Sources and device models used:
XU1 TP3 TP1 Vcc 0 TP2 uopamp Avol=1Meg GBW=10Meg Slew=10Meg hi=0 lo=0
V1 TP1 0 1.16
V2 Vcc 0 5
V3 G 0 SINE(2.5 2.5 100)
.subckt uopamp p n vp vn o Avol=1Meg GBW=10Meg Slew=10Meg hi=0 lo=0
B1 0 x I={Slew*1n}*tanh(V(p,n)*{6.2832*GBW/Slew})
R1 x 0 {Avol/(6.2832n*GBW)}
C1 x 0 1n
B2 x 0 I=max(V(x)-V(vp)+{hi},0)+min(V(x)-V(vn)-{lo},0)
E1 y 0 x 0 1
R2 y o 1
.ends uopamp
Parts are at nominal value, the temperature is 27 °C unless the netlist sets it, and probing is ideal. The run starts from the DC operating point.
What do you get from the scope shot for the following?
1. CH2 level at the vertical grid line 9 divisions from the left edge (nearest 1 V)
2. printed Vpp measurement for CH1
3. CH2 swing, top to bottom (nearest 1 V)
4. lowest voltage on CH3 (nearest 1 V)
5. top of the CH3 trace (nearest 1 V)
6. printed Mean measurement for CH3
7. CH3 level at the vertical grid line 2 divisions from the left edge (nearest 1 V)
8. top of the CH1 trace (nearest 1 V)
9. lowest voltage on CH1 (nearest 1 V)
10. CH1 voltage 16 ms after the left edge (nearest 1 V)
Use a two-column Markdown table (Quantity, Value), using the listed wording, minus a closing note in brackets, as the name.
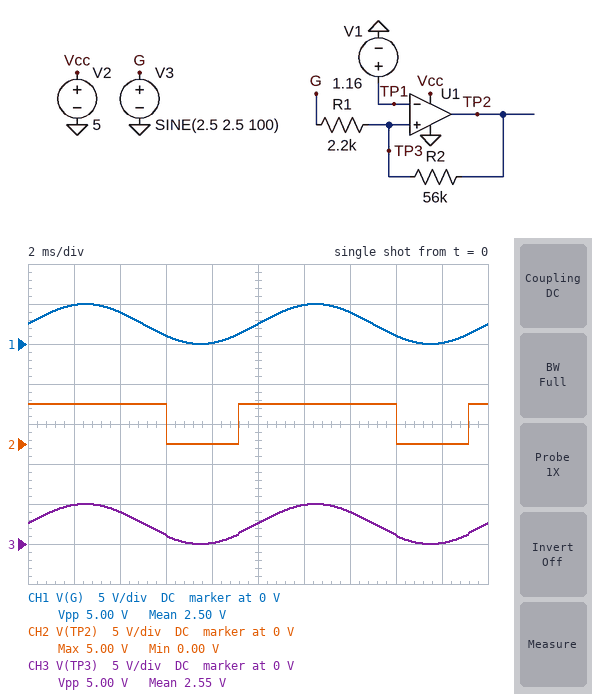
| Quantity | Value |
|---|---|
| CH2 level at the vertical grid line 9 divisions from the left edge | 0 V |
| printed Vpp measurement for CH1 | 5.00 V |
| CH2 swing, top to bottom | 5 V |
| lowest voltage on CH3 | 0 V |
| top of the CH3 trace | 5 V |
| printed Mean measurement for CH3 | 2.55 V |
| CH3 level at the vertical grid line 2 divisions from the left edge | 4 V |
| top of the CH1 trace | 5 V |
| lowest voltage on CH1 | 0 V |
| CH1 voltage 16 ms after the left edge | 1 V |
